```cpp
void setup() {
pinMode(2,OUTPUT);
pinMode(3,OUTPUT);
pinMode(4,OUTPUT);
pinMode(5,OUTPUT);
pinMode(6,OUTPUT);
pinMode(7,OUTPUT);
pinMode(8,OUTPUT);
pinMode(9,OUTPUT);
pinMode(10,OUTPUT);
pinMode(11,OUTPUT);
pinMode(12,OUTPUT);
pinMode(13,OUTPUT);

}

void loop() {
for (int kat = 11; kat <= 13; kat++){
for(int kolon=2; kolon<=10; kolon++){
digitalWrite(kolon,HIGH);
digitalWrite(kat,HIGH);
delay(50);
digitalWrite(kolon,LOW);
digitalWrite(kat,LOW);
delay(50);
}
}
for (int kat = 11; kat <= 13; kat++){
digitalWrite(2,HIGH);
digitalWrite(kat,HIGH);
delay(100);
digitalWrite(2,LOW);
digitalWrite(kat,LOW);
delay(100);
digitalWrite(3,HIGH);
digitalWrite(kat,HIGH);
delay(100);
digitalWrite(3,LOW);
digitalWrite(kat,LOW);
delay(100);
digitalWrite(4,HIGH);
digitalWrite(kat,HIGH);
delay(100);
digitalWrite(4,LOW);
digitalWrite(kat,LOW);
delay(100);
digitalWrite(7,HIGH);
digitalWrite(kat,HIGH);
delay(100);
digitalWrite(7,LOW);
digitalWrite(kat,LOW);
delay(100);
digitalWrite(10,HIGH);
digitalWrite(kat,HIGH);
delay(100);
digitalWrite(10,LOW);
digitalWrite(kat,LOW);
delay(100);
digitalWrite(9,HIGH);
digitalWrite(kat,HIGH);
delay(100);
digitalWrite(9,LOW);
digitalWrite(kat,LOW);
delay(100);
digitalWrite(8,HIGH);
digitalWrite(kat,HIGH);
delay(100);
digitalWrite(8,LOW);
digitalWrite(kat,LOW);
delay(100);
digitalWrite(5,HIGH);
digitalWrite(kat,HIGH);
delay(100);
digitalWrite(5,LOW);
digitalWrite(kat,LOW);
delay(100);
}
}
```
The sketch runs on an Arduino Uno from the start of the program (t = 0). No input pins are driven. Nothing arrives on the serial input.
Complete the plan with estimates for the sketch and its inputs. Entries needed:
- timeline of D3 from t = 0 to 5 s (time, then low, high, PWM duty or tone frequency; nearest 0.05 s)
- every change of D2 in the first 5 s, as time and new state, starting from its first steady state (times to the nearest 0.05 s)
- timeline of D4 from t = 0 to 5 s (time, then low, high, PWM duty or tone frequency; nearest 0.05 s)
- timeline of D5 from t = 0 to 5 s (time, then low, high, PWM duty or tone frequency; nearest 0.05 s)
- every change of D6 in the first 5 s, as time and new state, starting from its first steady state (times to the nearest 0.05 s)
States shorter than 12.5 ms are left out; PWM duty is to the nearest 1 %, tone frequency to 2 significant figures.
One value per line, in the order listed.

0 s low; 0.1 s high; 0.15 s low; 1 s high; 1.05 s low; 1.9 s high; 1.95 s low; 2.9 s high; 3 s low; 4.5 s high; 4.6 s low
0 s high; 0.05 s low; 0.9 s high; 0.95 s low; 1.8 s high; 1.85 s low; 2.7 s high; 2.8 s low; 4.3 s high; 4.4 s low
0 s low; 0.2 s high; 0.25 s low; 1.1 s high; 1.15 s low; 2 s high; 2.05 s low; 3.1 s high; 3.2 s low; 4.7 s high; 4.8 s low
0 s low; 0.3 s high; 0.35 s low; 1.2 s high; 1.25 s low; 2.1 s high; 2.15 s low; 4.1 s high; 4.2 s low
0 s low; 0.4 s high; 0.45 s low; 1.3 s high; 1.35 s low; 2.2 s high; 2.25 s low
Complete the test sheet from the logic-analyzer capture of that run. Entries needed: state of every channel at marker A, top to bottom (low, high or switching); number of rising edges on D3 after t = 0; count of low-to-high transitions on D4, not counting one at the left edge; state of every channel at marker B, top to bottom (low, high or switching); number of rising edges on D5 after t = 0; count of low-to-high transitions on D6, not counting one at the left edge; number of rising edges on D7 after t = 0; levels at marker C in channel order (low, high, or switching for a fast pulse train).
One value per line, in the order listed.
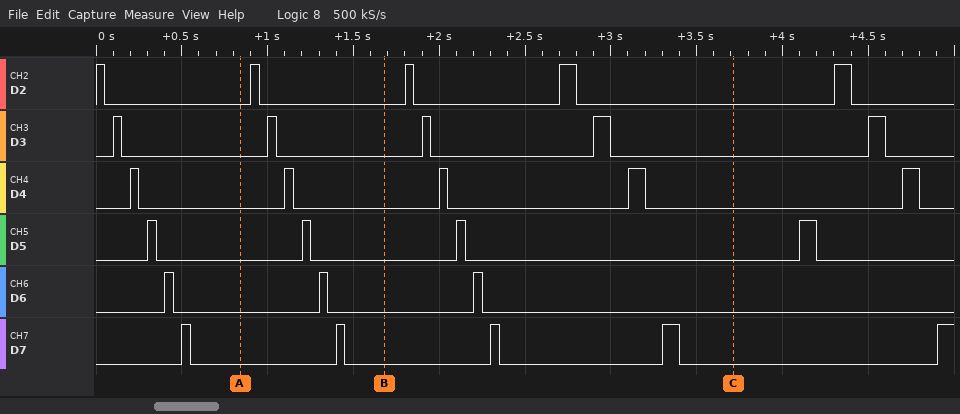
D2 low, D3 low, D4 low, D5 low, D6 low, D7 low
5
5
D2 low, D3 low, D4 low, D5 low, D6 low, D7 low
4
3
5
D2 low, D3 low, D4 low, D5 low, D6 low, D7 low
